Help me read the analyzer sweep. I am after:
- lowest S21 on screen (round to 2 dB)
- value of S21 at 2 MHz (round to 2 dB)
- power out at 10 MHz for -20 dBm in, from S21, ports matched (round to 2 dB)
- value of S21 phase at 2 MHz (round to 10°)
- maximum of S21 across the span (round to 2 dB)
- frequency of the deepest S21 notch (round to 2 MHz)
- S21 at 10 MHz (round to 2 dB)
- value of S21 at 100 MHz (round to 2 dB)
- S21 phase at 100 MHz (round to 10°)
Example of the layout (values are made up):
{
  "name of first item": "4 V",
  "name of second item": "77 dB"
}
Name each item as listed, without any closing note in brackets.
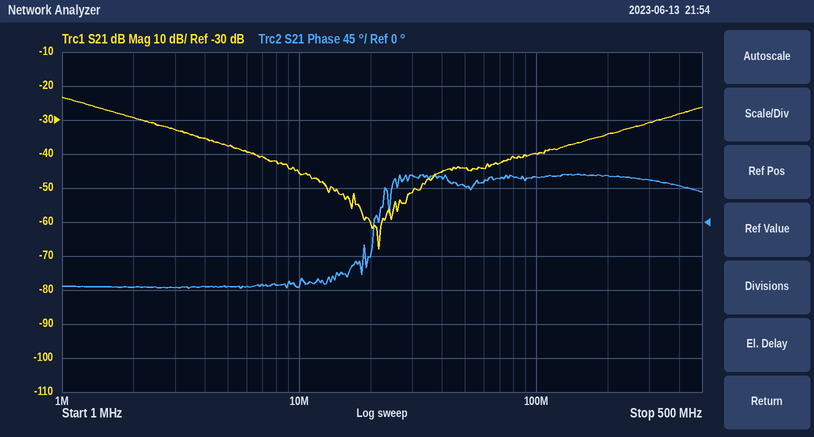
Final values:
{
  "lowest S21 on screen": "-68 dB",
  "value of S21 at 2 MHz": "-30 dB",
  "power out at 10 MHz for -20 dBm in, from S21, ports matched": "-66 dBm",
  "value of S21 phase at 2 MHz": "-90°",
  "maximum of S21 across the span": "-24 dB",
  "frequency of the deepest S21 notch": "22 MHz",
  "S21 at 10 MHz": "-46 dB",
  "value of S21 at 100 MHz": "-40 dB",
  "S21 phase at 100 MHz": "60°"
}
